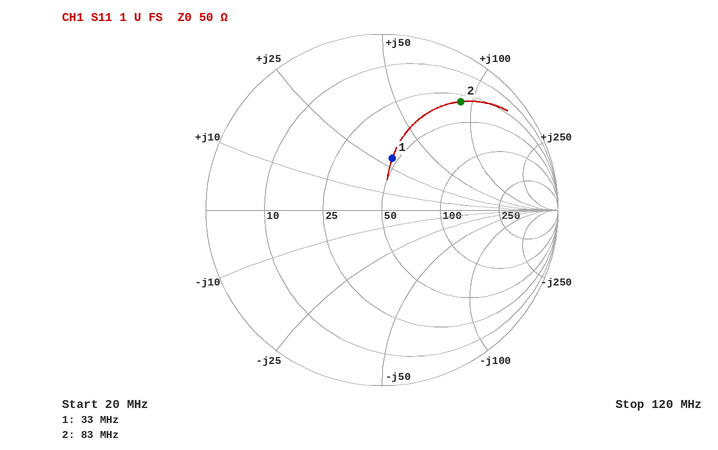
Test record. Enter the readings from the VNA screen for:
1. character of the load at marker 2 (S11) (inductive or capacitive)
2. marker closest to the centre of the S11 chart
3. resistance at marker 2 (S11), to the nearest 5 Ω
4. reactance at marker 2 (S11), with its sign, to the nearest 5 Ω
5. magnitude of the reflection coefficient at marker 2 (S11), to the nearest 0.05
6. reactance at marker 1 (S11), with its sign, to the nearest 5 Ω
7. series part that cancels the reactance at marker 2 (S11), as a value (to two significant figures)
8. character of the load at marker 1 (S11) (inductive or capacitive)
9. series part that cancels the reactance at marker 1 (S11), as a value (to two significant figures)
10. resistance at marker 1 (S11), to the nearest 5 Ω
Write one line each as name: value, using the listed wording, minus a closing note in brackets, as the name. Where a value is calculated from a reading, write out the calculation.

character of the load at marker 2 (S11): inductive
marker closest to the centre of the S11 chart: marker 1
resistance at marker 2 (S11), to the nearest 5 Ω: 30 Ω
reactance at marker 2 (S11), with its sign, to the nearest 5 Ω: +90 Ω
magnitude of the reflection coefficient at marker 2 (S11), to the nearest 0.05: 0.75
reactance at marker 1 (S11), with its sign, to the nearest 5 Ω: +30 Ω
series part that cancels the reactance at marker 2 (S11), as a value: C = 1/(2π × 83 MHz × 90 Ω) ≈ 21 pF
character of the load at marker 1 (S11): inductive
series part that cancels the reactance at marker 1 (S11), as a value: C = 1/(2π × 33 MHz × 30 Ω) ≈ 161 pF, so 160 pF to two significant figures
resistance at marker 1 (S11), to the nearest 5 Ω: 45 Ω
